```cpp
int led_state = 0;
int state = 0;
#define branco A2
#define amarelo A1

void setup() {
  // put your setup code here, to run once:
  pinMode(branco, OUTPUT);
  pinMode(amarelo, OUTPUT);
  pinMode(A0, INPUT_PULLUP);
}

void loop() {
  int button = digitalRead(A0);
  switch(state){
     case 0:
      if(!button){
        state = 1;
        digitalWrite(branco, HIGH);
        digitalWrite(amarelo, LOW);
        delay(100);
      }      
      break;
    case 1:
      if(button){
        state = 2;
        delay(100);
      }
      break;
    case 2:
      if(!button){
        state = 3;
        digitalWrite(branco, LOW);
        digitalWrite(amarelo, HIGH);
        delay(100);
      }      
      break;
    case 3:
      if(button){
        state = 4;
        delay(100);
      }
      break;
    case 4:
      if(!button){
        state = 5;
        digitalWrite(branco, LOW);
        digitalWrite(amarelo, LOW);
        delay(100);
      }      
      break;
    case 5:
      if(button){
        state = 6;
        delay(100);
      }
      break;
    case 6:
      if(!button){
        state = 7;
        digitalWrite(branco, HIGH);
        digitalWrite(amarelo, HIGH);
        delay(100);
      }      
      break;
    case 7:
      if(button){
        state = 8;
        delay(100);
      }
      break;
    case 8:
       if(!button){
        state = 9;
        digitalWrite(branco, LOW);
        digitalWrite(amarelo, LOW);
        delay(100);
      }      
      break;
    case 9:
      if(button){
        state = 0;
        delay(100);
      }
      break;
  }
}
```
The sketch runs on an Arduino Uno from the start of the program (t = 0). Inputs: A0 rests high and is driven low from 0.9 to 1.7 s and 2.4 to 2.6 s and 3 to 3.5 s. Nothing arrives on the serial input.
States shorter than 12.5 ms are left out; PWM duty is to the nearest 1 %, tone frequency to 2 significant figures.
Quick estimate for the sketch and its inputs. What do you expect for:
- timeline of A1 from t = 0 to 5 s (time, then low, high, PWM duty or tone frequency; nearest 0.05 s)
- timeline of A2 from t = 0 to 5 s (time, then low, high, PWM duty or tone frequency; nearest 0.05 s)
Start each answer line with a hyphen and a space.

- 0 s low; 2.4 s high; 3 s low
- 0 s low; 0.9 s high; 2.4 s low
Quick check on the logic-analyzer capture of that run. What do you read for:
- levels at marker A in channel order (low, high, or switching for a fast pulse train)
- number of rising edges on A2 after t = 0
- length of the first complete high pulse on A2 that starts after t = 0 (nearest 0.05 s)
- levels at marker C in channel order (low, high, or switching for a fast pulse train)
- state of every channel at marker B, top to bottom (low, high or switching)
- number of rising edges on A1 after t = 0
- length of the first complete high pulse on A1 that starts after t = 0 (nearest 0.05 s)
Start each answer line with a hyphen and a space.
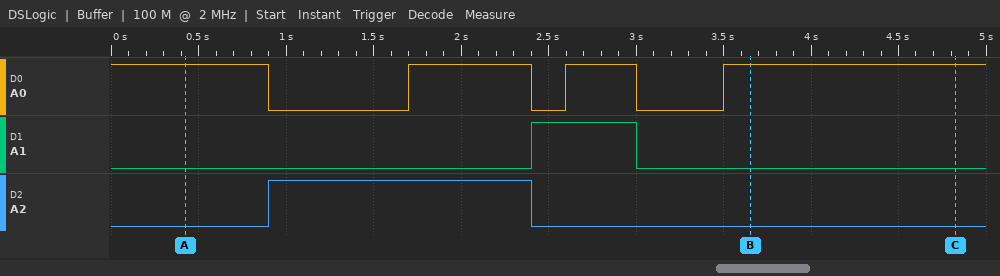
- A0 high, A1 low, A2 low
- 1
- 1.50 s
- A0 high, A1 low, A2 low
- A0 high, A1 low, A2 low
- 1
- 0.60 s
